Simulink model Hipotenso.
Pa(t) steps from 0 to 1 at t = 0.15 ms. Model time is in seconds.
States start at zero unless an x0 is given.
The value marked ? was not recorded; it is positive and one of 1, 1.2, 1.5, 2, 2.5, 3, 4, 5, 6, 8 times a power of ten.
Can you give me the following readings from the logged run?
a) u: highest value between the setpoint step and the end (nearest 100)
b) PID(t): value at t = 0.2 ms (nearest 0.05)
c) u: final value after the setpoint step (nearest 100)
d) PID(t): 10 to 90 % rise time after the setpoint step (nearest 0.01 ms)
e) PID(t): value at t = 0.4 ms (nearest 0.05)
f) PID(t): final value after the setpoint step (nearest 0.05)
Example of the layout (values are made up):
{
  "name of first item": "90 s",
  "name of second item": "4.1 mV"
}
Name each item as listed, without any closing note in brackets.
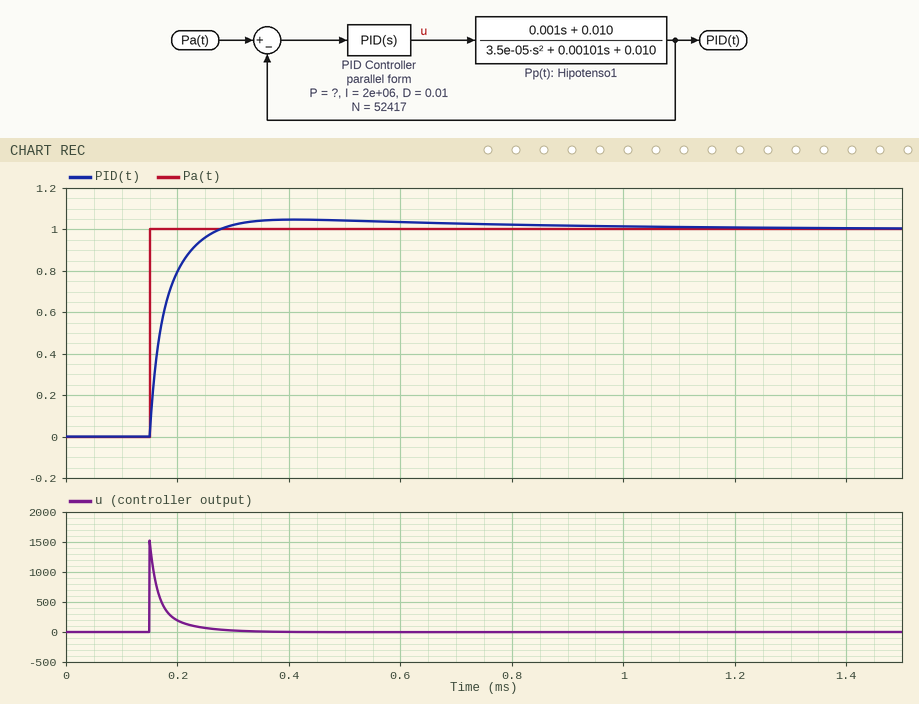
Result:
{
  "u: highest value between the setpoint step and the end": "1500",
  "PID(t): value at t = 0.2 ms": "0.80",
  "u: final value after the setpoint step": "0",
  "PID(t): 10 to 90 % rise time after the setpoint step": "0.07 ms",
  "PID(t): value at t = 0.4 ms": "1.05",
  "PID(t): final value after the setpoint step": "1.00"
}
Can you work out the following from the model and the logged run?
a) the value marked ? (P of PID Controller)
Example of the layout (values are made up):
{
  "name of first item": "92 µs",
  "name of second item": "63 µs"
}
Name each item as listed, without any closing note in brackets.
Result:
{
  "the value marked ?": "1000"
}
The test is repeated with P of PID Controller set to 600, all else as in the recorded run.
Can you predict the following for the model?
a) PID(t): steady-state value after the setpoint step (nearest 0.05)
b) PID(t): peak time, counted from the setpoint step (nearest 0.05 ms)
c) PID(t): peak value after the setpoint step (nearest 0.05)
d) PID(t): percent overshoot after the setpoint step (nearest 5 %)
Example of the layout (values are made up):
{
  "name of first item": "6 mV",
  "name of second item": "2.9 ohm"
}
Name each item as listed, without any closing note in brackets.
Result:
{
  "PID(t): steady-state value after the setpoint step": "1.00",
  "PID(t): peak time, counted from the setpoint step": "0.30 ms",
  "PID(t): peak value after the setpoint step": "1.10",
  "PID(t): percent overshoot after the setpoint step": "10 %"
}
